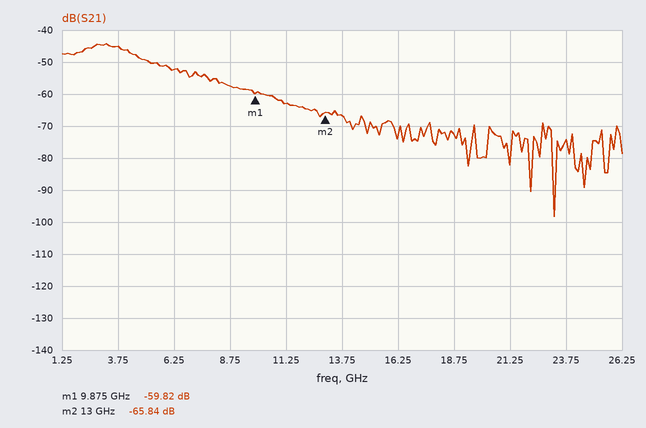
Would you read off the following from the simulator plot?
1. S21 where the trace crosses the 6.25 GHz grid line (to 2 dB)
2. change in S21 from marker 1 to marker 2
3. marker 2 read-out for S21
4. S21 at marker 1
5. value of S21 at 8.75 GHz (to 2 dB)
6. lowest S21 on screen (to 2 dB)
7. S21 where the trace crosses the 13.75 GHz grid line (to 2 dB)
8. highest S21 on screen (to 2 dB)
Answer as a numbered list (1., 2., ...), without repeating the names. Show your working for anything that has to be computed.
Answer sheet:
1. -52 dB
2. -65.84 − (-59.82) = -6.02 dB
3. -65.84 dB
4. -59.82 dB
5. -58 dB
6. -98 dB
7. -66 dB
8. -44 dB
